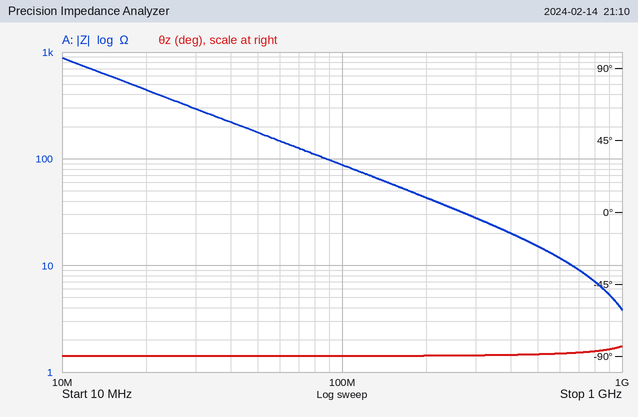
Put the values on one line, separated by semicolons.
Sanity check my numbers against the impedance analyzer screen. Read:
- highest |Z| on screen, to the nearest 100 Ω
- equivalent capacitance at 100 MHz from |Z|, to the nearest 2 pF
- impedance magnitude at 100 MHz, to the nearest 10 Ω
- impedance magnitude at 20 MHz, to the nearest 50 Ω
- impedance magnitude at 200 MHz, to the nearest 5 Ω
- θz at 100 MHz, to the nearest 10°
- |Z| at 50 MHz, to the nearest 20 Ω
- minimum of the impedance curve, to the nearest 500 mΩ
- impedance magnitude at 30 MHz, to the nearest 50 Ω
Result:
900 Ω; 18 pF; 90 Ω; 450 Ω; 45 Ω; -90°; 180 Ω; 4.0 Ω; 300 Ω
